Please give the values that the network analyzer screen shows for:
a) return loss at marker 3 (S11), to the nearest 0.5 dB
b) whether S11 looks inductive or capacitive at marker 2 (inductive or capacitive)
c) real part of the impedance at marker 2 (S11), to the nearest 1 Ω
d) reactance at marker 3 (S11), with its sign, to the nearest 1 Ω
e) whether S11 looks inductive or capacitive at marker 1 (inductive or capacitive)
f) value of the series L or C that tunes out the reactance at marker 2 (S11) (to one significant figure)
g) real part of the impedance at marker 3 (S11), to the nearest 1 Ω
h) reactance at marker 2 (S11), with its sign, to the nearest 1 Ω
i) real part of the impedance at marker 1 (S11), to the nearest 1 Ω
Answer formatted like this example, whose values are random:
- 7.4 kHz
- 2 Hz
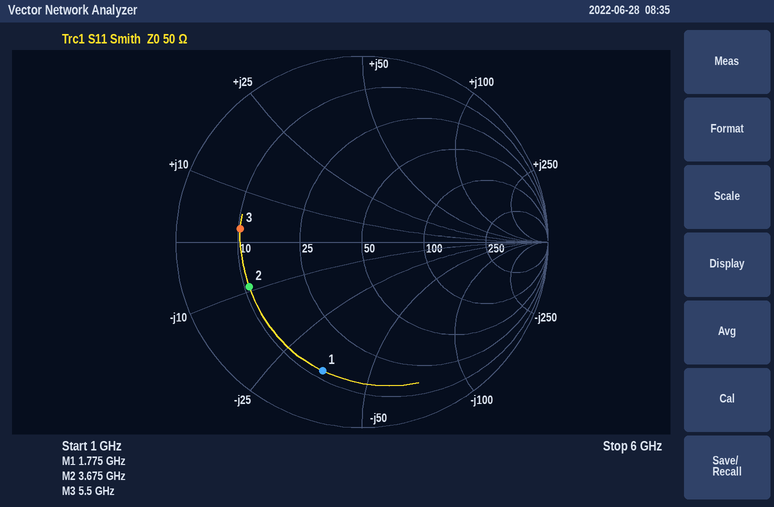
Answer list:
- 3.5 dB
- capacitive
- 11 Ω
- +3 Ω
- capacitive
- 400 pH
- 10 Ω
- -9 Ω
- 12 Ω
